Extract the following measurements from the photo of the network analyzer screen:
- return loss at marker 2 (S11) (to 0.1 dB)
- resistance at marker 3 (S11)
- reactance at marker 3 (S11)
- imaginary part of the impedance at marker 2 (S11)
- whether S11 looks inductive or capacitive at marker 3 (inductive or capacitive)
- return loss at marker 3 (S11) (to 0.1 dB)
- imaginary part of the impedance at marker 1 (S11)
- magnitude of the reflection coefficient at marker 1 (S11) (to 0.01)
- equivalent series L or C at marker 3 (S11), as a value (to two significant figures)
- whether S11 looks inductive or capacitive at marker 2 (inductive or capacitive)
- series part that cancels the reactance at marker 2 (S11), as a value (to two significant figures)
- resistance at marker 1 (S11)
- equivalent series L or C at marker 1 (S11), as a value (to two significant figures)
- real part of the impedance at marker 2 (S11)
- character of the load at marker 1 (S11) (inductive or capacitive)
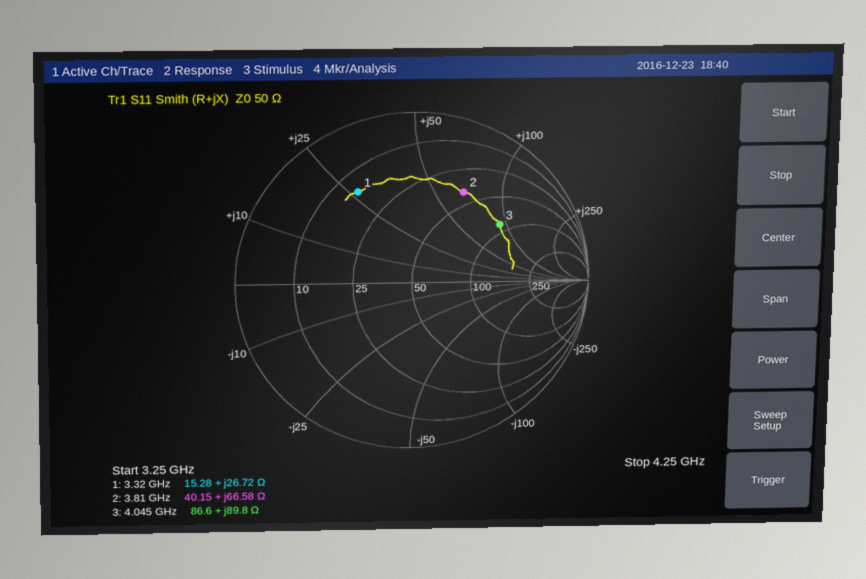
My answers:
4.4 dB
86.6 Ω
+89.8 Ω
+66.58 Ω
inductive
4.5 dB
+26.72 Ω
0.62
3.5 nH
inductive
630 fF
15.28 Ω
1.3 nH
40.15 Ω
inductive
